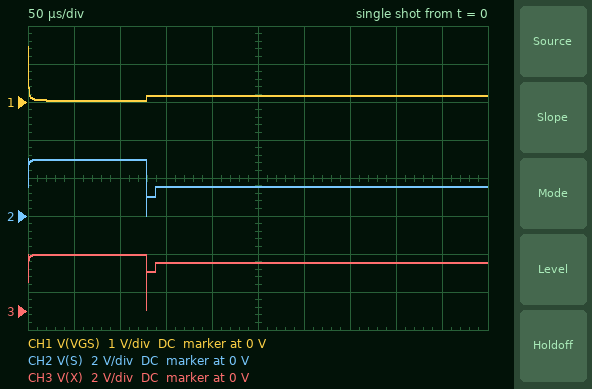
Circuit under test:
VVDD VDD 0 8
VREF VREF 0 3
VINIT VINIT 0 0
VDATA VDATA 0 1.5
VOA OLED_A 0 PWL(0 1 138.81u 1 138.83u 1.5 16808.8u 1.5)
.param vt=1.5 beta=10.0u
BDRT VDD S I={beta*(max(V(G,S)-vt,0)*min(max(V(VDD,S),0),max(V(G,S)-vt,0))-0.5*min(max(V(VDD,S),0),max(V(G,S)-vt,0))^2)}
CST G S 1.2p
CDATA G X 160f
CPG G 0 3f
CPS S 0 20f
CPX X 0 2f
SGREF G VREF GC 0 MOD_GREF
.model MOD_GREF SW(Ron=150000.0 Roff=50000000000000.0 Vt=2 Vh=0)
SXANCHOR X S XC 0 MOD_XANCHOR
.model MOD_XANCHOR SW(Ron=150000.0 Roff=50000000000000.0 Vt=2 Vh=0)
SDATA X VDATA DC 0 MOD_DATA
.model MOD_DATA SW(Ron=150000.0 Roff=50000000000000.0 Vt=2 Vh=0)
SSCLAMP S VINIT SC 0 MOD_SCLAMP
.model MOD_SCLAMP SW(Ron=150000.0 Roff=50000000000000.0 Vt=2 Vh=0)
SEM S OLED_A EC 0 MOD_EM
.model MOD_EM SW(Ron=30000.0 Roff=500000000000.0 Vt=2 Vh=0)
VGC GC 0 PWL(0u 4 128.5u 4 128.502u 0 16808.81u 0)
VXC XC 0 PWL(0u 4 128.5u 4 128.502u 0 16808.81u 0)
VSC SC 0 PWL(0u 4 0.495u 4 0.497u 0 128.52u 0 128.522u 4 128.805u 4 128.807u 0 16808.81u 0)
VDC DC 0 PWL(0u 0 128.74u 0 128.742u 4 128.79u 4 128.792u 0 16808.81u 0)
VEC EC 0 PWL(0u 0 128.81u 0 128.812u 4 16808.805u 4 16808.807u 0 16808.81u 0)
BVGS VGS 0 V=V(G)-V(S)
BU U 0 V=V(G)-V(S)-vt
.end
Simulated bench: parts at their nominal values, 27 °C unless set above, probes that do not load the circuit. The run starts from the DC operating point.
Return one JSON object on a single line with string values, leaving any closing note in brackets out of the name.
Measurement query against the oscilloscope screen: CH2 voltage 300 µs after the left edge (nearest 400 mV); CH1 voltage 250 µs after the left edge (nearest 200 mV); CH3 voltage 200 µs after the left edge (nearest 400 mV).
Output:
{"CH2 voltage 300 µs after the left edge": "1.6 V", "CH1 voltage 250 µs after the left edge": "200 mV", "CH3 voltage 200 µs after the left edge": "2.4 V"}
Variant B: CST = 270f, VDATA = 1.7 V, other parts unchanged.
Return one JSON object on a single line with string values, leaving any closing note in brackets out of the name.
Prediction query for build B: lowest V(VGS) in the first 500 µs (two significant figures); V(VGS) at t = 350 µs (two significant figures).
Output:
{"lowest V(VGS) in the first 500 µs": "27 mV", "V(VGS) at t = 350 µs": "500 mV"}
